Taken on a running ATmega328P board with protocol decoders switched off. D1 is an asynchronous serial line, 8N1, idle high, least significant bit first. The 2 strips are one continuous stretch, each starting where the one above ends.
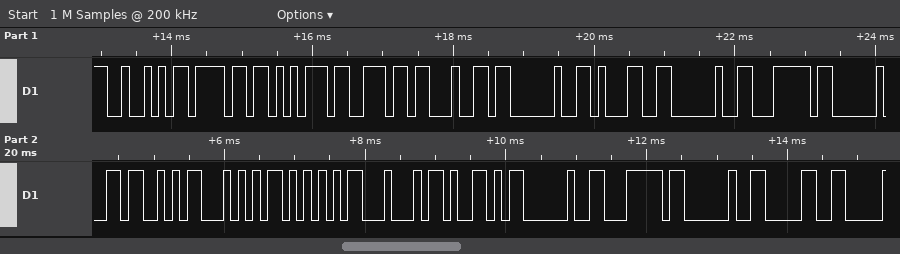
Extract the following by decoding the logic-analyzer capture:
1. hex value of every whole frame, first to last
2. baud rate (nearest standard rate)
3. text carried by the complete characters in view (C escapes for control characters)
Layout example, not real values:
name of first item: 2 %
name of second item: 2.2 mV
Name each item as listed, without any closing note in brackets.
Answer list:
hex value of every whole frame, first to last: 52 6F 75 6E 64 20 31 20 7C 20 53 54 55 44 59 20 7C 20 30
baud rate: 9600 baud
text carried by the complete characters in view: "Round 1 | STUDY | 0"
